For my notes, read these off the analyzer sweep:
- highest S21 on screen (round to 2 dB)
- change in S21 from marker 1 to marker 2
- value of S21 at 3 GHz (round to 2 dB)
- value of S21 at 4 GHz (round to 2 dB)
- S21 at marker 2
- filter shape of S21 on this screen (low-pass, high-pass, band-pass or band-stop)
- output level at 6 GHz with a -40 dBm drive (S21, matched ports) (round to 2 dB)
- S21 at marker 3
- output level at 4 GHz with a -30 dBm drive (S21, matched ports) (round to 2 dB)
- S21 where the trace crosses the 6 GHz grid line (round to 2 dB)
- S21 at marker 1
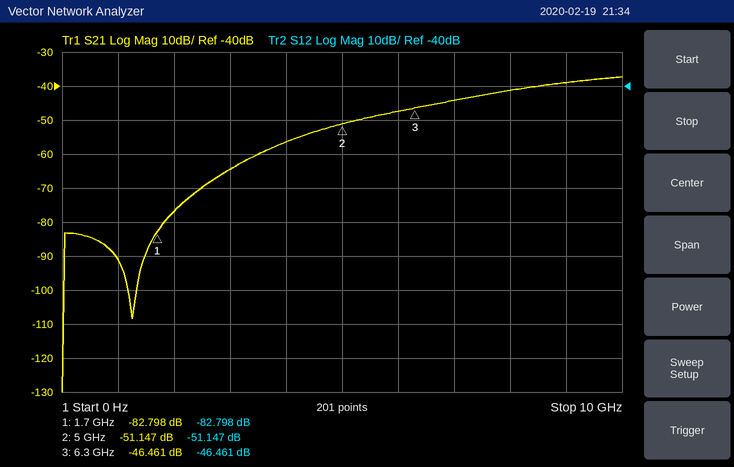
-38 dB
31.651 dB
-64 dB
-56 dB
-51.147 dB
high-pass
-88 dBm
-46.461 dB
-86 dBm
-48 dB
-82.798 dB
